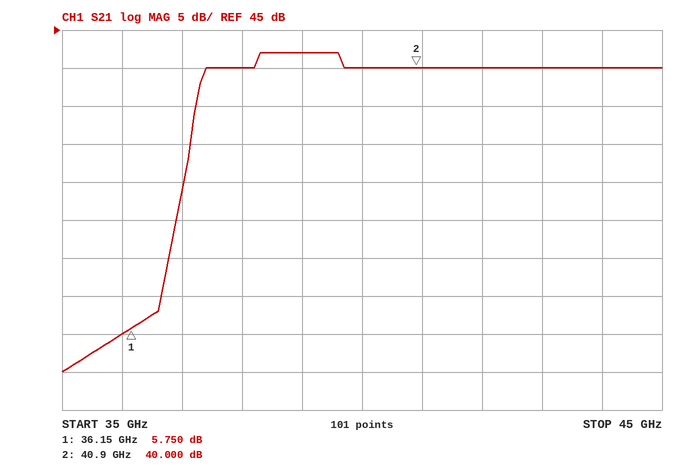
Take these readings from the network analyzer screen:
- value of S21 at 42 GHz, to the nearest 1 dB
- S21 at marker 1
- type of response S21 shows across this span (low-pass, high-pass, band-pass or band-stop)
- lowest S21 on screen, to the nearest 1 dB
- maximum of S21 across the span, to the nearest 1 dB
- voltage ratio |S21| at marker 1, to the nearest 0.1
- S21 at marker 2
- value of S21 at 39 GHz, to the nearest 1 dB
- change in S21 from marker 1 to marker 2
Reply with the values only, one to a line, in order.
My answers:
40 dB
5.750 dB
high-pass
0 dB
42 dB
1.9
40.000 dB
42 dB
34.250 dB
